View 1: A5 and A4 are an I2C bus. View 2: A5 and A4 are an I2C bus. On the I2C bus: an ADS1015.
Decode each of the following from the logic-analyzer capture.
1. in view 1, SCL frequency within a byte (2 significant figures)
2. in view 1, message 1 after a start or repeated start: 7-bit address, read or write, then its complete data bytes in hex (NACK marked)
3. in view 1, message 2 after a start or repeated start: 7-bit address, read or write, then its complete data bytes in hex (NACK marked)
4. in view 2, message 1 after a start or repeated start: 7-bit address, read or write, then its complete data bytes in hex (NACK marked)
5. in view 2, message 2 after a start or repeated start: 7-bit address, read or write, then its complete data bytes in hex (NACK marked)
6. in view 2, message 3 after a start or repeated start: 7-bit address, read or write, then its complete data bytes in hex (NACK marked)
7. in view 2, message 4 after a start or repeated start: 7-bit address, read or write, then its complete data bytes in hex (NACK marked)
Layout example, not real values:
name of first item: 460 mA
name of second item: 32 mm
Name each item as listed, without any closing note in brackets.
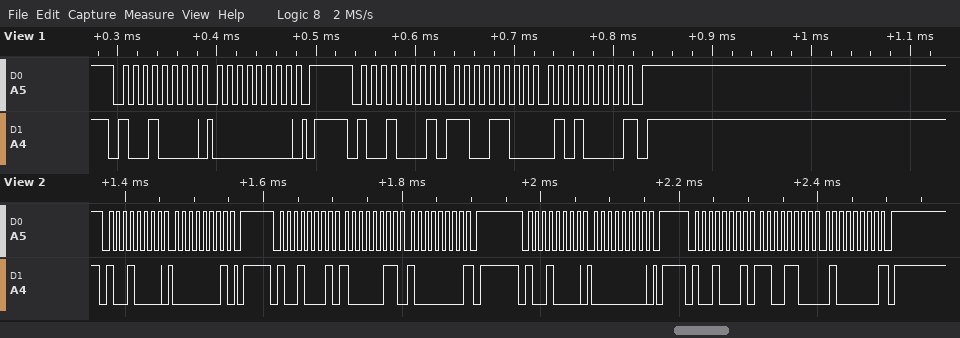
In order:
in view 1, SCL frequency within a byte: 100 kHz
in view 1, message 1 after a start or repeated start: 7-bit address, read or write, then its complete data bytes in hex: 0x48 write: 00
in view 1, message 2 after a start or repeated start: 7-bit address, read or write, then its complete data bytes in hex: 0x48 read: CC 50 NACK
in view 2, message 1 after a start or repeated start: 7-bit address, read or write, then its complete data bytes in hex: 0x48 write: 01
in view 2, message 2 after a start or repeated start: 7-bit address, read or write, then its complete data bytes in hex: 0x48 read: 83 80 NACK
in view 2, message 3 after a start or repeated start: 7-bit address, read or write, then its complete data bytes in hex: 0x48 write: 00
in view 2, message 4 after a start or repeated start: 7-bit address, read or write, then its complete data bytes in hex: 0x48 read: CC 40 NACK
